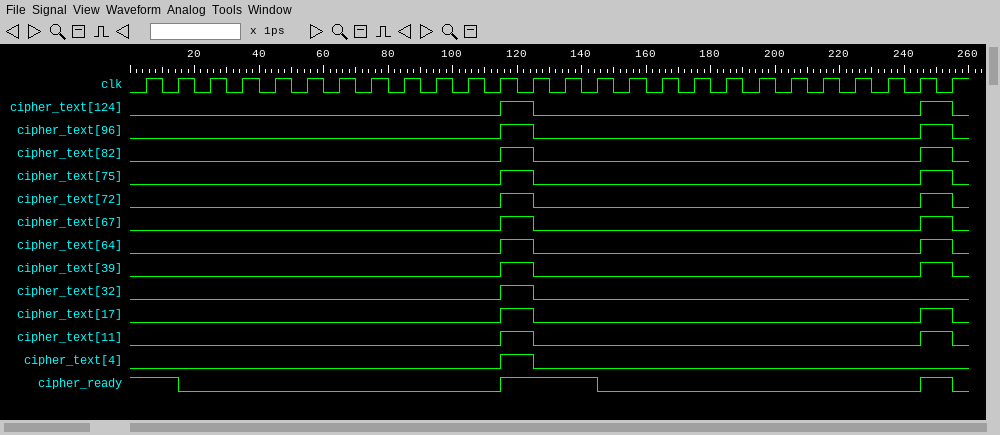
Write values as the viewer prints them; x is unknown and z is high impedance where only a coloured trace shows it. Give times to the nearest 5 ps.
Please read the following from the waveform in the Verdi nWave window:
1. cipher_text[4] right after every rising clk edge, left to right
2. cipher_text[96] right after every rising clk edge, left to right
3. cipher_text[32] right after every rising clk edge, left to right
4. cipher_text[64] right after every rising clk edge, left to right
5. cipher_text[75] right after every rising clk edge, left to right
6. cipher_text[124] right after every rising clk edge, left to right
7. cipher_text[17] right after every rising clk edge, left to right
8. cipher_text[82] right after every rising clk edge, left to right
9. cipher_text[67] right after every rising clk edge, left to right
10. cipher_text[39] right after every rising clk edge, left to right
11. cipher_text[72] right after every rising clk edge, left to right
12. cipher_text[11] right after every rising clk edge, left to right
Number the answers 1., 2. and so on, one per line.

1. 0 0 0 0 0 0 0 0 0 0 0 1 0 0 0 0 0 0 0 0 0 0 0 0 0 0
2. 0 0 0 0 0 0 0 0 0 0 0 1 0 0 0 0 0 0 0 0 0 0 0 0 1 0
3. 0 0 0 0 0 0 0 0 0 0 0 1 0 0 0 0 0 0 0 0 0 0 0 0 0 0
4. 0 0 0 0 0 0 0 0 0 0 0 1 0 0 0 0 0 0 0 0 0 0 0 0 1 0
5. 0 0 0 0 0 0 0 0 0 0 0 1 0 0 0 0 0 0 0 0 0 0 0 0 1 0
6. 0 0 0 0 0 0 0 0 0 0 0 1 0 0 0 0 0 0 0 0 0 0 0 0 1 0
7. 0 0 0 0 0 0 0 0 0 0 0 1 0 0 0 0 0 0 0 0 0 0 0 0 1 0
8. 0 0 0 0 0 0 0 0 0 0 0 1 0 0 0 0 0 0 0 0 0 0 0 0 1 0
9. 0 0 0 0 0 0 0 0 0 0 0 1 0 0 0 0 0 0 0 0 0 0 0 0 1 0
10. 0 0 0 0 0 0 0 0 0 0 0 1 0 0 0 0 0 0 0 0 0 0 0 0 1 0
11. 0 0 0 0 0 0 0 0 0 0 0 1 0 0 0 0 0 0 0 0 0 0 0 0 1 0
12. 0 0 0 0 0 0 0 0 0 0 0 1 0 0 0 0 0 0 0 0 0 0 0 0 1 0
